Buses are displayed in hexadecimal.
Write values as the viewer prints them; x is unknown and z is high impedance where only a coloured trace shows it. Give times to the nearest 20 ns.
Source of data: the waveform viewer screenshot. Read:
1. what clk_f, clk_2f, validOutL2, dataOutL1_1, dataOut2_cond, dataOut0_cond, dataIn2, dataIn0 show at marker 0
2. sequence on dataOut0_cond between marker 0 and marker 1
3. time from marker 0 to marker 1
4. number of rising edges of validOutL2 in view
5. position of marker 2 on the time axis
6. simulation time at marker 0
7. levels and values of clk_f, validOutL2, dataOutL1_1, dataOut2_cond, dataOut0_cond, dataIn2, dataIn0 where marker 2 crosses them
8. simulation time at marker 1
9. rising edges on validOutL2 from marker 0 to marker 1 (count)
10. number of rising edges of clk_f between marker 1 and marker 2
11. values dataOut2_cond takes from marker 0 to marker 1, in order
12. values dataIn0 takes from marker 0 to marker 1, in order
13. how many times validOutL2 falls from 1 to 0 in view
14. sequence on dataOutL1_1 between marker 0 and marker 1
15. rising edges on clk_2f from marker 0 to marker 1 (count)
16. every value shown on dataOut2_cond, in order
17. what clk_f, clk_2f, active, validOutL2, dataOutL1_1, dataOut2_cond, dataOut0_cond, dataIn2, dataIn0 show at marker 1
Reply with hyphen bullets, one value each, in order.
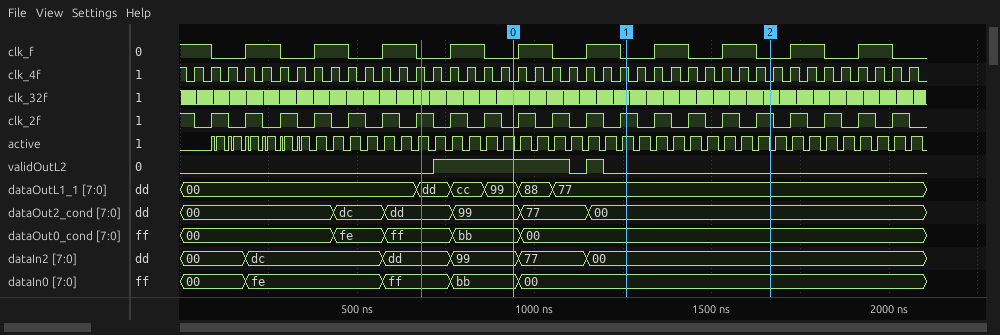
- clk_f=0, clk_2f=0, validOutL2=1, dataOutL1_1=99, dataOut2_cond=99, dataOut0_cond=bb, dataIn2=99, dataIn0=bb
- bb, 00
- 320 ns
- 2
- 1660 ns
- 940 ns
- clk_f=0, validOutL2=0, dataOutL1_1=77, dataOut2_cond=00, dataOut0_cond=00, dataIn2=00, dataIn0=00
- 1260 ns
- 1
- 2
- 99, 77, 00
- bb, 00
- 2
- 99, 88, 77
- 4
- 00, dc, dd, 99, 77, 00
- clk_f=0, clk_2f=1, active=1, validOutL2=0, dataOutL1_1=77, dataOut2_cond=00, dataOut0_cond=00, dataIn2=00, dataIn0=00
